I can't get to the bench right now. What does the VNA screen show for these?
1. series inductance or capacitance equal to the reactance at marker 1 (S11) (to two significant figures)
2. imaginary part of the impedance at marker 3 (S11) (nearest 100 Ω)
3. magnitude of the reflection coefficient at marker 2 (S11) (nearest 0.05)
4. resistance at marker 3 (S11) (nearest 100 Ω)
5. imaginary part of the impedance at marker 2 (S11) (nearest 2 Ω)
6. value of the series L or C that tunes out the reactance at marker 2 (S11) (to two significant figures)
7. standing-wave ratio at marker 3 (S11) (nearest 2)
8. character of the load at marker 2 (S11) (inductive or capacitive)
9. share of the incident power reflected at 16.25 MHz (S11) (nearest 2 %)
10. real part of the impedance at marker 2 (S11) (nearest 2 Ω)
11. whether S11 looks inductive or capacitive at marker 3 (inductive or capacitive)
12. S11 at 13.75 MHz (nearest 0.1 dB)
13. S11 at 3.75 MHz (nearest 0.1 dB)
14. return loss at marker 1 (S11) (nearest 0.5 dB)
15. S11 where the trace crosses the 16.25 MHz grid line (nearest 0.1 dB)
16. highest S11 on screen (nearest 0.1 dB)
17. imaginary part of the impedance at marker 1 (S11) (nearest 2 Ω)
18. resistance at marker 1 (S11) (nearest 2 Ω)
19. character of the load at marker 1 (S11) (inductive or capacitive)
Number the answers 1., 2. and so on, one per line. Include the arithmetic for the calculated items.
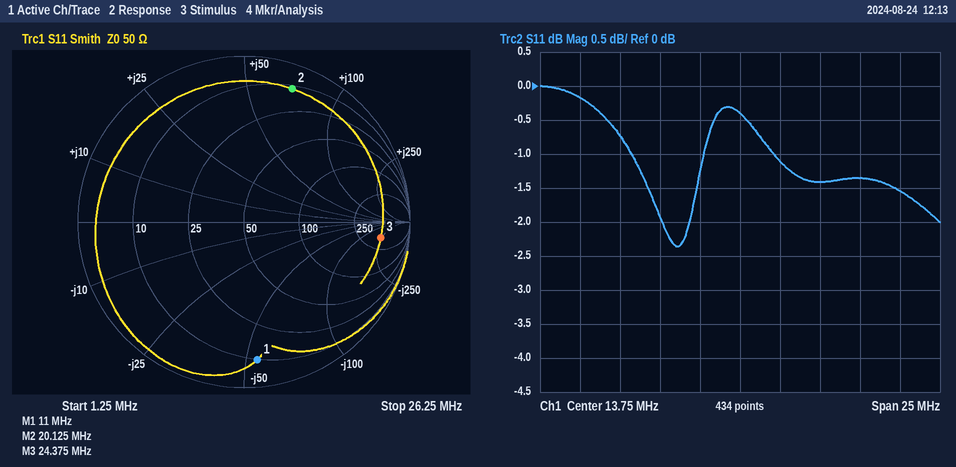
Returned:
1. C = 1/(2π × 11 MHz × 54 Ω) ≈ 268 pF, so 270 pF to two significant figures
2. -200 Ω
3. 0.85
4. 400 Ω
5. +70 Ω
6. C = 1/(2π × 20.125 MHz × 70 Ω) ≈ 113 pF, so 110 pF to two significant figures
7. 10
8. inductive
9. 10^(-1.1/10) ≈ 78 %
10. 12 Ω
11. capacitive
12. -0.4 dB
13. -0.2 dB
14. 1.5 dB
15. -1.1 dB
16. 0.0 dB
17. -54 Ω
18. 10 Ω
19. capacitive
